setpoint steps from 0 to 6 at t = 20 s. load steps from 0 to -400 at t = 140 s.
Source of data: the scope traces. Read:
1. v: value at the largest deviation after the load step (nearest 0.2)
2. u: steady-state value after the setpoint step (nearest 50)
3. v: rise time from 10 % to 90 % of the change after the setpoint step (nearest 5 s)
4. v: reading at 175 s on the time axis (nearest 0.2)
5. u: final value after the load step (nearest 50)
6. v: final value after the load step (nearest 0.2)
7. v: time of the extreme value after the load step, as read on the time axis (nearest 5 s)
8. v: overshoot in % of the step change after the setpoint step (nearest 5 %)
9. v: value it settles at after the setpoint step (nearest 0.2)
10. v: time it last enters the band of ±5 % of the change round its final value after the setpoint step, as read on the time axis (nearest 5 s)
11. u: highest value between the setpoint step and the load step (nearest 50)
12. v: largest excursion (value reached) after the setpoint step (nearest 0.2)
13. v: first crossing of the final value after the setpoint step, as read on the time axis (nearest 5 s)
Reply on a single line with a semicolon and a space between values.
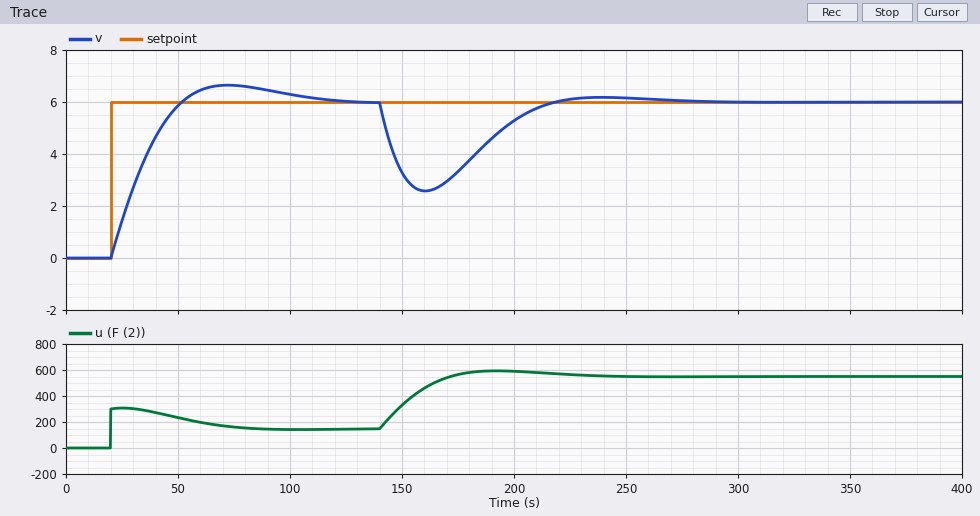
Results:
2.6; 150; 25 s; 3.4; 550; 6.0; 160 s; 10 %; 6.0; 100 s; 300; 6.6; 50 s
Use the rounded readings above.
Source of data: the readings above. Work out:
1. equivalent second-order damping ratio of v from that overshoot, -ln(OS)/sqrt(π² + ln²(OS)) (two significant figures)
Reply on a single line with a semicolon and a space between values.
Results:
0.59
